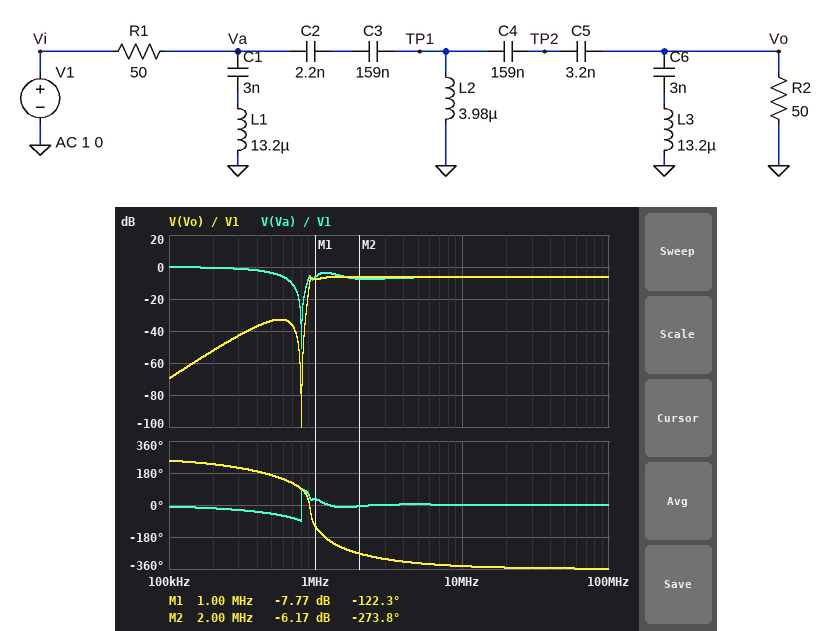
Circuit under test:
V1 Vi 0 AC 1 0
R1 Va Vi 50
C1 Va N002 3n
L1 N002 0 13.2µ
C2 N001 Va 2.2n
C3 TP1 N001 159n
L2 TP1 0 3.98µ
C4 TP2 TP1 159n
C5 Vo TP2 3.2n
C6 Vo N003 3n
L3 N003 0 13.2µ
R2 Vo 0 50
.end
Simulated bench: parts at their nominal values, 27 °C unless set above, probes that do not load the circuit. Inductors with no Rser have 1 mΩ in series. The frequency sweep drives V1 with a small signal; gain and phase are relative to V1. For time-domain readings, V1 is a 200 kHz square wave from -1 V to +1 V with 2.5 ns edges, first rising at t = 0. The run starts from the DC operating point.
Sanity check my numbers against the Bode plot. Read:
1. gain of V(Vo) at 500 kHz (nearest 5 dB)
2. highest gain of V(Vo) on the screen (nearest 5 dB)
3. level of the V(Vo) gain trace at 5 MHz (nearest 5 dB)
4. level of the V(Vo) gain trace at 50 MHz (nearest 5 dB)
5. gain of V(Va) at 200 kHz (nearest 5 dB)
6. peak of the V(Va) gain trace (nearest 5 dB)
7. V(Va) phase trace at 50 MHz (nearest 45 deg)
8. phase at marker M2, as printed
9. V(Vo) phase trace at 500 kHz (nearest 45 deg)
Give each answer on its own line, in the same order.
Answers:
-35 dB
-5 dB
-5 dB
-5 dB
0 dB
0 dB
0 deg
-273.8 deg
180 deg
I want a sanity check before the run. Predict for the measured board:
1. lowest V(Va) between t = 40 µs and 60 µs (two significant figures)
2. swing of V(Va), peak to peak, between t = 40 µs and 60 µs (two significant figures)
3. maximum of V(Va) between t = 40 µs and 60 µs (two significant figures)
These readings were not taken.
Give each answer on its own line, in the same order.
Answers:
-1.2 V
2.3 V
1.2 V
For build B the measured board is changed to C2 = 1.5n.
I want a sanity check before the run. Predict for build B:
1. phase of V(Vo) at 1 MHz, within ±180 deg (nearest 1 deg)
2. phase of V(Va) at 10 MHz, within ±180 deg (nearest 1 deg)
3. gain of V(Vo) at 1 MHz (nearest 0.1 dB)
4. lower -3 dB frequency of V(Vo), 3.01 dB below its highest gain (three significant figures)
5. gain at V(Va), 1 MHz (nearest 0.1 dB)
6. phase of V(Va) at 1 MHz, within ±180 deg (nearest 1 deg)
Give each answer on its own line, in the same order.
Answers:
-96 deg
0 deg
-9.8 dB
1.13 MHz
-4.9 dB
41 deg
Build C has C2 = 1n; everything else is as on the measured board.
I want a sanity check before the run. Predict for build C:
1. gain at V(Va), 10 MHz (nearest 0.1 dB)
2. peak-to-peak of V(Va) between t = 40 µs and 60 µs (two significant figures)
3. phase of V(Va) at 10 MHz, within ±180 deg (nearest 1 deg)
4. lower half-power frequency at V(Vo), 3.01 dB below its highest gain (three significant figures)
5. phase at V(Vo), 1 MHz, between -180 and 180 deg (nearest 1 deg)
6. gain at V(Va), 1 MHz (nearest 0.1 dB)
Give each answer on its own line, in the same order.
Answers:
-6.0 dB
2.5 V
-3 deg
1.54 MHz
-76 deg
-4.8 dB
